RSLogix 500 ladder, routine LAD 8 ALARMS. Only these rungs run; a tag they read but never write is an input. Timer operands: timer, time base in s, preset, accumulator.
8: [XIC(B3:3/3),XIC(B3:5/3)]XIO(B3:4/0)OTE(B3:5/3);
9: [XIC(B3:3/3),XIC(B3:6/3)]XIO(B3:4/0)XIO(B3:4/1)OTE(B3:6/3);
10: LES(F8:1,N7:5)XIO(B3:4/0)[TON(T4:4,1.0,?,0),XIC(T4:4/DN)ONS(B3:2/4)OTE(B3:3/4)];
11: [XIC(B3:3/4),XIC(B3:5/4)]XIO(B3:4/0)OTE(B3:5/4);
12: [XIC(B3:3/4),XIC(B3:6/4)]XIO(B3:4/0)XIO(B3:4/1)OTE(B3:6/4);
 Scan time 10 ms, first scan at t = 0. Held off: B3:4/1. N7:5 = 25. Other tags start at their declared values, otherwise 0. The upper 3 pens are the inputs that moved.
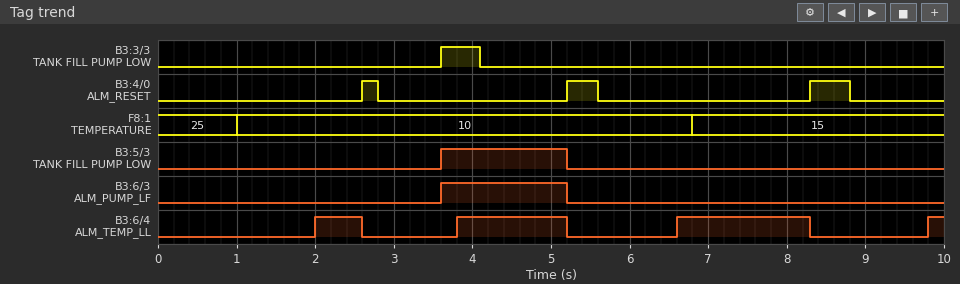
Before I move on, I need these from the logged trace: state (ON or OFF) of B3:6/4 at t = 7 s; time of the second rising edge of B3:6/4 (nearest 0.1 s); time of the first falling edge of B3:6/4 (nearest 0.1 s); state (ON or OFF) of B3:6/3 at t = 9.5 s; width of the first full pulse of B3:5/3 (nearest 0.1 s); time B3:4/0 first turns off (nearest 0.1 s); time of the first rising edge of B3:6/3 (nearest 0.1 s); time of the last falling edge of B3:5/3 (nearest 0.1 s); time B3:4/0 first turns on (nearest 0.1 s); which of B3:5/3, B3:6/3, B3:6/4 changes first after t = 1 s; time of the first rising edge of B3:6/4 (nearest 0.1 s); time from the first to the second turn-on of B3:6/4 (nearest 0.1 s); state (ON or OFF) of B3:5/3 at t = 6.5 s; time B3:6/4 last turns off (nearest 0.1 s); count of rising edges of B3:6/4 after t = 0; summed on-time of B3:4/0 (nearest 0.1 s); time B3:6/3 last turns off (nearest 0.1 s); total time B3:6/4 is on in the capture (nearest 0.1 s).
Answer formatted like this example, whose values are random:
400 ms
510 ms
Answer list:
ON
3.8 s
2.6 s
OFF
1.6 s
2.8 s
3.6 s
5.2 s
2.6 s
B3:6/4
2.0 s
1.8 s
OFF
8.3 s
4
1.1 s
5.2 s
3.9 s
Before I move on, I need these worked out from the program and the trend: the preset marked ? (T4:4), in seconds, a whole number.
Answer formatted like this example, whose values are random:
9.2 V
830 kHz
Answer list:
1 s
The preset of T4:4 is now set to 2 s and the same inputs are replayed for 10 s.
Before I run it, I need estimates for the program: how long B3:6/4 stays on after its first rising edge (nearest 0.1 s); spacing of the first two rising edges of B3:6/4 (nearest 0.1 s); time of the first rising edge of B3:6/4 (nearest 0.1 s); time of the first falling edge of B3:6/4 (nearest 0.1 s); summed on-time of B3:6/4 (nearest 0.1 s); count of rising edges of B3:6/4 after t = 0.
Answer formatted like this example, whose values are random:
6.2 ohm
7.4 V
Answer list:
0.4 s
2.8 s
4.8 s
5.2 s
1.1 s
2
